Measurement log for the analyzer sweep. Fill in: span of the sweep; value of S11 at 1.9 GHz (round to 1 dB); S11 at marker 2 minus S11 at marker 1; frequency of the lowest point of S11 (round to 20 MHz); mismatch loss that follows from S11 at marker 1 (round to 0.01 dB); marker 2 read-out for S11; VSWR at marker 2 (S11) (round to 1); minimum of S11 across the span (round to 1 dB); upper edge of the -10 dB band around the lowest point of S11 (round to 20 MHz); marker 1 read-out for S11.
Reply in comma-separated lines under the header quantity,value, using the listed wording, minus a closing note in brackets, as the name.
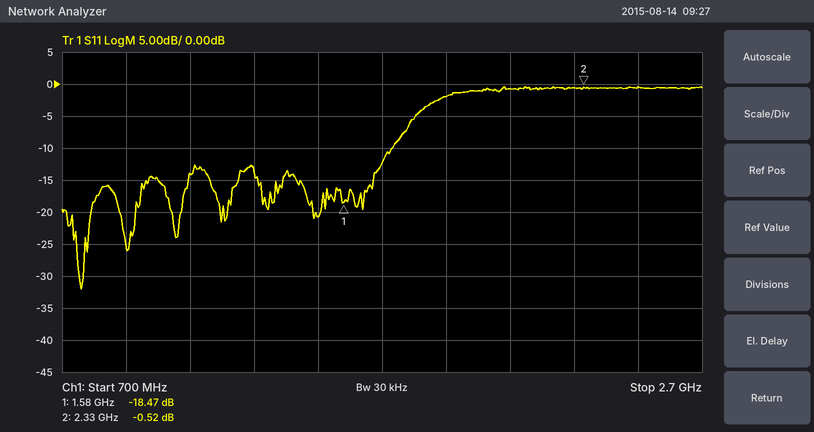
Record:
quantity,value
span of the sweep,2 GHz
value of S11 at 1.9 GHz,-2 dB
S11 at marker 2 minus S11 at marker 1,17.95 dB
frequency of the lowest point of S11,760 MHz
mismatch loss that follows from S11 at marker 1,0.06 dB
marker 2 read-out for S11,-0.52 dB
VSWR at marker 2 (S11),33
minimum of S11 across the span,-32 dB
upper edge of the -10 dB band around the lowest point of S11,1.74 GHz
marker 1 read-out for S11,-18.47 dB
